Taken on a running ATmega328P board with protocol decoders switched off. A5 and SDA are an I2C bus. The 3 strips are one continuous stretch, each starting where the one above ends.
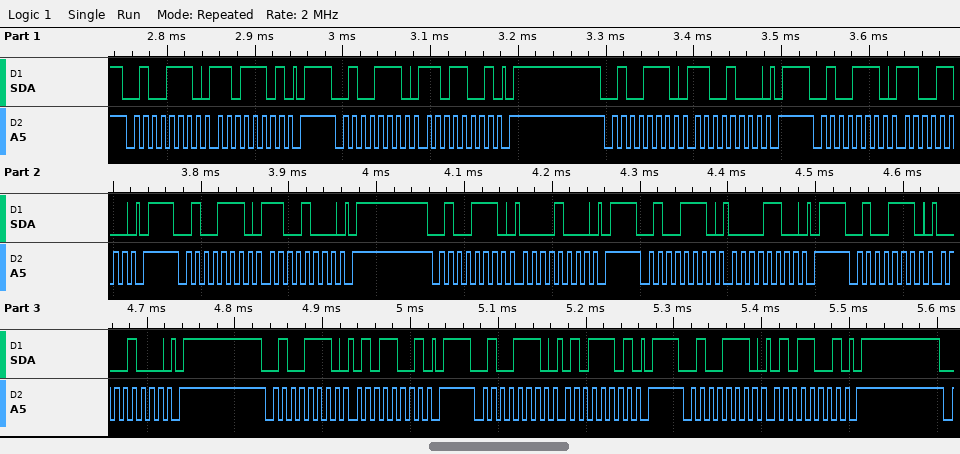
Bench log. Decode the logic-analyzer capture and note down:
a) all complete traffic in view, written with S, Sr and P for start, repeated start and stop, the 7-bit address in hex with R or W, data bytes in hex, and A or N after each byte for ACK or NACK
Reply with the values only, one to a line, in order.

S 27W A DD A P S 27W A D9 A P S 27W A C8 A P S 27W A CC A P S 27W A C8 A P S 27W A 08 A P S 27W A 0C A P S 27W A 08 A P S 27W A 59 A P S 27W A 5D A P S 27W A 59 A P
